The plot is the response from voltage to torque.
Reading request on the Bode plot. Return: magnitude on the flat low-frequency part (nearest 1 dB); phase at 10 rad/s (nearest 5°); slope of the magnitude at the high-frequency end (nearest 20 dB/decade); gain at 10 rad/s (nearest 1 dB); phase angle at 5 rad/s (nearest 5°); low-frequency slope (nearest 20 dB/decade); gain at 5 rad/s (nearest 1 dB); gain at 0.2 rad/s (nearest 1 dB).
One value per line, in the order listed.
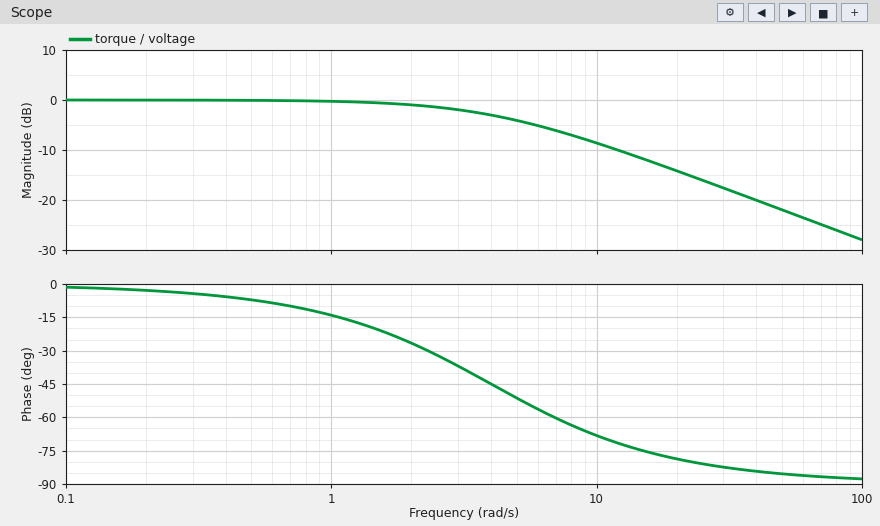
0 dB
-70°
-20 dB/decade
-9 dB
-50°
0 dB/decade
-4 dB
0 dB
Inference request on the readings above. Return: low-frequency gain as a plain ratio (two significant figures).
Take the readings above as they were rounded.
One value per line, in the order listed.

1.0
